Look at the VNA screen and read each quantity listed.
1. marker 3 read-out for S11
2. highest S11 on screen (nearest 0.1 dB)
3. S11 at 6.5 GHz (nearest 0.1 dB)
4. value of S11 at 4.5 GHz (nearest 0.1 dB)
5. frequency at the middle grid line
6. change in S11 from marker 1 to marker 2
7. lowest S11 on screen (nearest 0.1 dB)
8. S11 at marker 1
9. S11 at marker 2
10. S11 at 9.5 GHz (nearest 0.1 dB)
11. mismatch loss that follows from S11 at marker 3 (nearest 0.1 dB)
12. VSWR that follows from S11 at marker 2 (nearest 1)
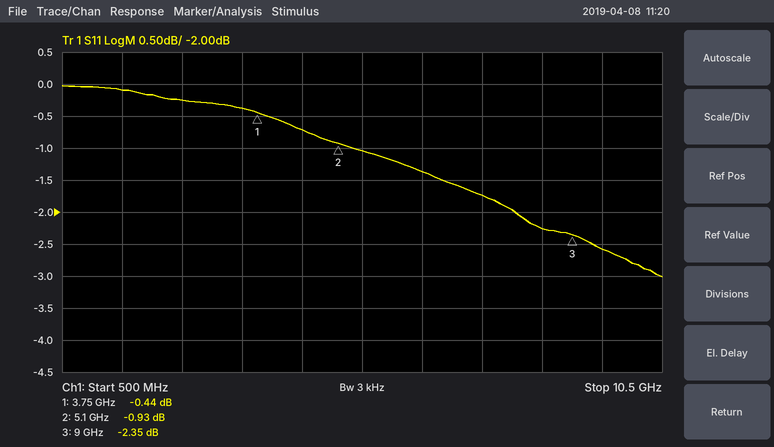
-2.35 dB
0.0 dB
-1.4 dB
-0.7 dB
5.5 GHz
-0.49 dB
-3.0 dB
-0.44 dB
-0.93 dB
-2.6 dB
3.8 dB
19
